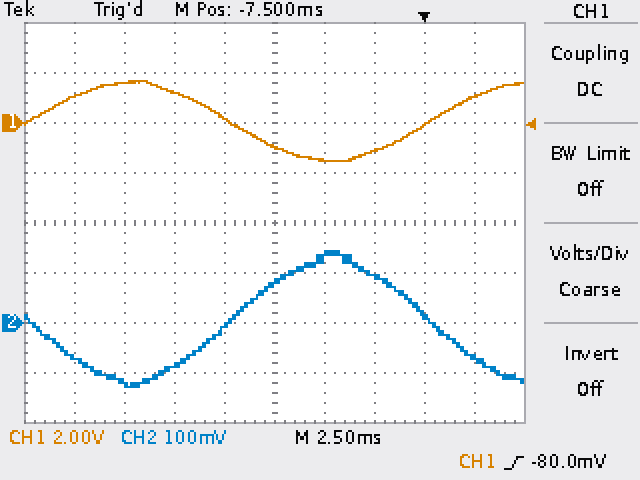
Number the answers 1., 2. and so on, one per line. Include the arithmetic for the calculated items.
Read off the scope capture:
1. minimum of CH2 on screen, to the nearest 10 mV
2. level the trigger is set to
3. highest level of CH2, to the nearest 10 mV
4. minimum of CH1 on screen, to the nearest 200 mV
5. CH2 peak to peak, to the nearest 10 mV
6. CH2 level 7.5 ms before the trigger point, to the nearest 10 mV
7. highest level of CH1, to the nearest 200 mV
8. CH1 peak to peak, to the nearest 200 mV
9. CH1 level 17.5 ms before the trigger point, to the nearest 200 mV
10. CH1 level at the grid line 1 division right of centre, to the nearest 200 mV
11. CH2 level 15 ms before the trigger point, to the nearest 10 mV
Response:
1. -130 mV
2. -80.0 mV
3. 140 mV
4. -1.6 V
5. 140 mV − (-130 mV) = 270 mV
6. 80 mV
7. 1.6 V
8. 1.6 V − (-1.6 V) = 3.2 V
9. 1.0 V
10. -1.4 V
11. -120 mV
